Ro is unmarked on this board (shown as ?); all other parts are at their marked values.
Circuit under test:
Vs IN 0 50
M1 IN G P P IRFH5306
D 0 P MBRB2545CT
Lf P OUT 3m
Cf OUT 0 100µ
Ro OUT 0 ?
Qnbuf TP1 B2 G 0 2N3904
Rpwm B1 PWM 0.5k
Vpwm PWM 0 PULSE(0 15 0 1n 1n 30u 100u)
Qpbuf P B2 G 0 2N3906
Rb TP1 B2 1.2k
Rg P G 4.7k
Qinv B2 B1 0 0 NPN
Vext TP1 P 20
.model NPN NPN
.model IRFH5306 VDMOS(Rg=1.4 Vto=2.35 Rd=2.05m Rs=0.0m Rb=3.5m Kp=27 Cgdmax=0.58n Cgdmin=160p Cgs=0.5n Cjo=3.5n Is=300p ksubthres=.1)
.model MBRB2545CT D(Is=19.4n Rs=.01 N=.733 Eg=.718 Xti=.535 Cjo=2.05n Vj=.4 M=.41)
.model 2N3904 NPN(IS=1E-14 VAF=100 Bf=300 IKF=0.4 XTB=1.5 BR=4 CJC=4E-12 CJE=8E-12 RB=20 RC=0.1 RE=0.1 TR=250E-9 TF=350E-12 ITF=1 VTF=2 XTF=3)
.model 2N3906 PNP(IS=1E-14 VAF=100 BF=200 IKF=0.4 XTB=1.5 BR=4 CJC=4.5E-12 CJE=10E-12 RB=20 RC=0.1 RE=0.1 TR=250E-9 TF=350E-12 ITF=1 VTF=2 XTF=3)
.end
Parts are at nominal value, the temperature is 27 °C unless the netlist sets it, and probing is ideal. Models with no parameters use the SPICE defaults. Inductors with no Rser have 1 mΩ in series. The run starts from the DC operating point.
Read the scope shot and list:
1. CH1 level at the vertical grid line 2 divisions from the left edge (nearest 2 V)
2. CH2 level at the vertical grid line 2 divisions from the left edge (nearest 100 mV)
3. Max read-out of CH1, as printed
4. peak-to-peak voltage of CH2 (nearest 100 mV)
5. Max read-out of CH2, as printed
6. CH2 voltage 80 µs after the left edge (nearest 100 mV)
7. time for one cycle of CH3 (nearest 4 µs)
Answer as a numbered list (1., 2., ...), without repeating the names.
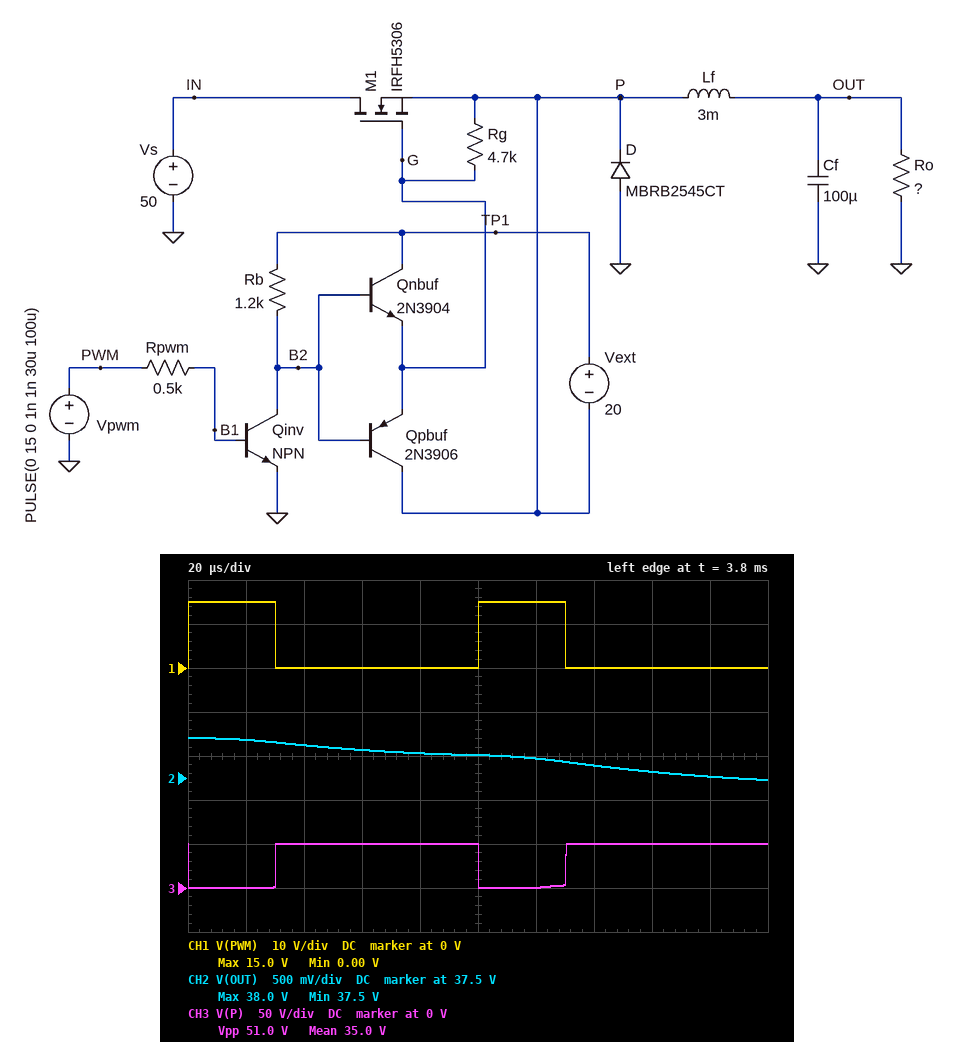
1. 0 V
2. 37.9 V
3. 15.0 V
4. 500 mV
5. 38.0 V
6. 37.8 V
7. 100 µs
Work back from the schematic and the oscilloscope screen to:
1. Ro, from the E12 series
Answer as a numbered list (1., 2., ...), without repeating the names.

1. 120 Ω
